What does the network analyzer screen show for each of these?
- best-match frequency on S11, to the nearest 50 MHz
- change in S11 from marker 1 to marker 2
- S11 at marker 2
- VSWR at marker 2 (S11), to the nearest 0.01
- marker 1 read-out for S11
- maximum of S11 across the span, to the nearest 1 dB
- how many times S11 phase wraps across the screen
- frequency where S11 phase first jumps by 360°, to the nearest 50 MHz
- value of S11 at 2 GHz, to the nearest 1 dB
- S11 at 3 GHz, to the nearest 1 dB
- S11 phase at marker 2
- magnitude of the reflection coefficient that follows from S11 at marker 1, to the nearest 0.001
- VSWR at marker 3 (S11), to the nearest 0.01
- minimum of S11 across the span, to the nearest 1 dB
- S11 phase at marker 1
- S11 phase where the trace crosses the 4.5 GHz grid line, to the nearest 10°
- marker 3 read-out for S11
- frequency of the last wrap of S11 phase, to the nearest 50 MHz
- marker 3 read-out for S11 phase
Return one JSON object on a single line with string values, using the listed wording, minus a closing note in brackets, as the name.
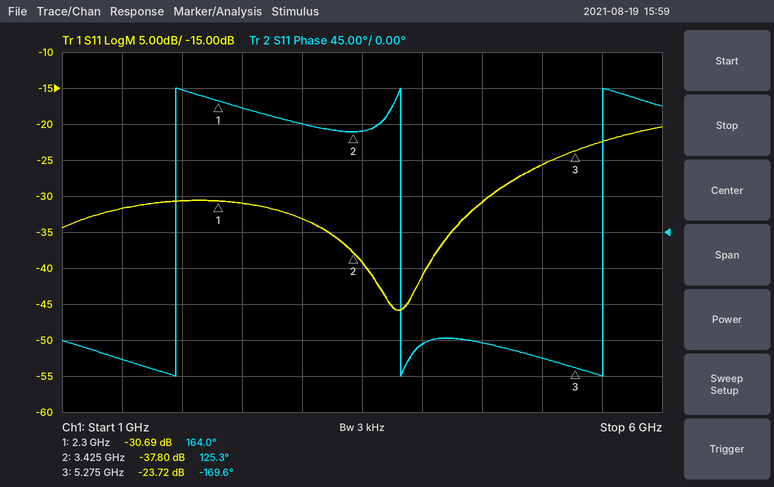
{"best-match frequency on S11, to the nearest 50 MHz": "3.80 GHz", "change in S11 from marker 1 to marker 2": "-7.11 dB", "S11 at marker 2": "-37.80 dB", "VSWR at marker 2 (S11), to the nearest 0.01": "1.03", "marker 1 read-out for S11": "-30.69 dB", "maximum of S11 across the span, to the nearest 1 dB": "-20 dB", "how many times S11 phase wraps across the screen": "3", "frequency where S11 phase first jumps by 360°, to the nearest 50 MHz": "1.95 GHz", "value of S11 at 2 GHz, to the nearest 1 dB": "-31 dB", "S11 at 3 GHz, to the nearest 1 dB": "-33 dB", "S11 phase at marker 2": "125.3°", "magnitude of the reflection coefficient that follows from S11 at marker 1, to the nearest 0.001": "0.029", "VSWR at marker 3 (S11), to the nearest 0.01": "1.14", "minimum of S11 across the span, to the nearest 1 dB": "-46 dB", "S11 phase at marker 1": "164.0°", "S11 phase where the trace crosses the 4.5 GHz grid line, to the nearest 10°": "-140°", "marker 3 read-out for S11": "-23.72 dB", "frequency of the last wrap of S11 phase, to the nearest 50 MHz": "5.50 GHz", "marker 3 read-out for S11 phase": "-169.6°"}
